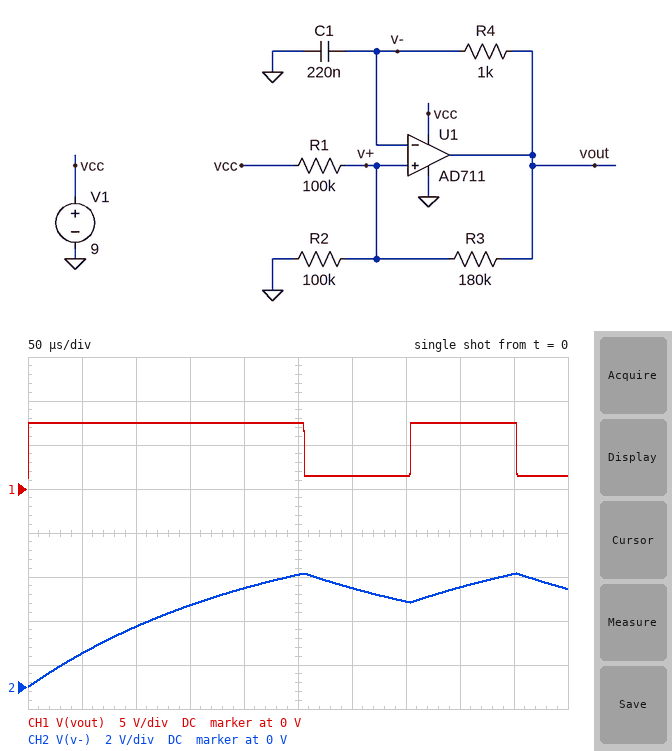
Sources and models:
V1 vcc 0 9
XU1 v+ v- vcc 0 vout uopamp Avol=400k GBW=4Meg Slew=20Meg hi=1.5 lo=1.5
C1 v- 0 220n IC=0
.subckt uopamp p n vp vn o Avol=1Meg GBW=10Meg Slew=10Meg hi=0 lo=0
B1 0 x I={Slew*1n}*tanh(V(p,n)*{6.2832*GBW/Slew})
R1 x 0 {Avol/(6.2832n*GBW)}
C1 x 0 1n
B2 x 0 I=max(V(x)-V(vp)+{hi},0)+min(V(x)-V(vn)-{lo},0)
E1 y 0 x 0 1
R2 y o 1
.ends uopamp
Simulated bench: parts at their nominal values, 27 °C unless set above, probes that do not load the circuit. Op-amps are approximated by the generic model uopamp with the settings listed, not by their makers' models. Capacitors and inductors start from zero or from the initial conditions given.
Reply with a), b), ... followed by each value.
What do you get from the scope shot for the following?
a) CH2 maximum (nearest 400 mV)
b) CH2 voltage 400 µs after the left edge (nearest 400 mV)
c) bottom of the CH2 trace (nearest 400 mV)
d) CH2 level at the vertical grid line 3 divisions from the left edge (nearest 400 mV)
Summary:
a) 5.2 V
b) 4.4 V
c) 0 V
d) 3.6 V
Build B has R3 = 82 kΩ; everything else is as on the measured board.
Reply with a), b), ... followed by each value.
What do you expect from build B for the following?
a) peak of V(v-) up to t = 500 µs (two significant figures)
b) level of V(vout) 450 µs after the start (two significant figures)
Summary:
a) 5.6 V
b) 1.5 V
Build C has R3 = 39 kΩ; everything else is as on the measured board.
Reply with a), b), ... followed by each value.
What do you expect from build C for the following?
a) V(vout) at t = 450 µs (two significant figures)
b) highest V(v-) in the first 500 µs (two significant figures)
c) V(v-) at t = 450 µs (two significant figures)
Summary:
a) 1.5 V
b) 6.2 V
c) 4.9 V
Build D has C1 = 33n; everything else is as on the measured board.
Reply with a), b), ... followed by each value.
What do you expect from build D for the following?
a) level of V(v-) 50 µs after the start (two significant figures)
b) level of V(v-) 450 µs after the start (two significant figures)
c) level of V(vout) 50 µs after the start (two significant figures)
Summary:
a) 4.1 V
b) 4.6 V
c) 1.5 V
